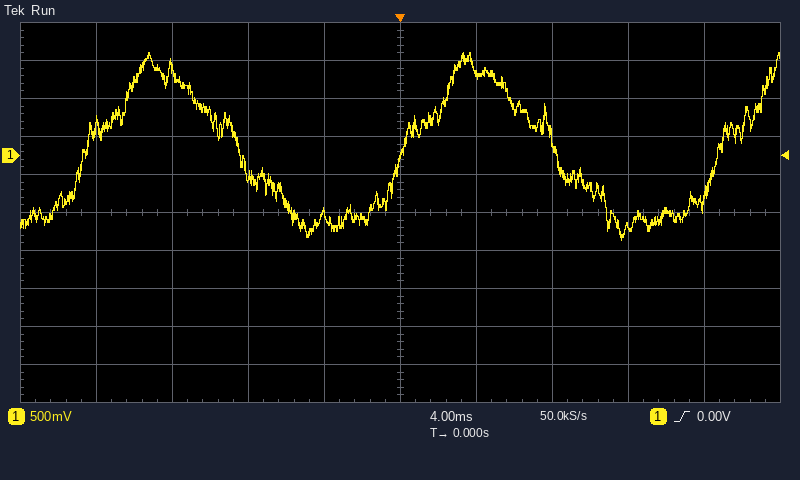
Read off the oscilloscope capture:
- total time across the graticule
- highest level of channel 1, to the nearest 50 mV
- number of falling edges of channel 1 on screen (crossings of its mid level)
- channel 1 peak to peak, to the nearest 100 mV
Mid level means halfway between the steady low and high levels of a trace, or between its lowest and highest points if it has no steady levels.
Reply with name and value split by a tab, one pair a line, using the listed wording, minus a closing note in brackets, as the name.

total time across the graticule	40 ms
highest level of channel 1, to the nearest 50 mV	1.35 V
number of falling edges of channel 1 on screen	2
channel 1 peak to peak, to the nearest 100 mV	2.50 V
